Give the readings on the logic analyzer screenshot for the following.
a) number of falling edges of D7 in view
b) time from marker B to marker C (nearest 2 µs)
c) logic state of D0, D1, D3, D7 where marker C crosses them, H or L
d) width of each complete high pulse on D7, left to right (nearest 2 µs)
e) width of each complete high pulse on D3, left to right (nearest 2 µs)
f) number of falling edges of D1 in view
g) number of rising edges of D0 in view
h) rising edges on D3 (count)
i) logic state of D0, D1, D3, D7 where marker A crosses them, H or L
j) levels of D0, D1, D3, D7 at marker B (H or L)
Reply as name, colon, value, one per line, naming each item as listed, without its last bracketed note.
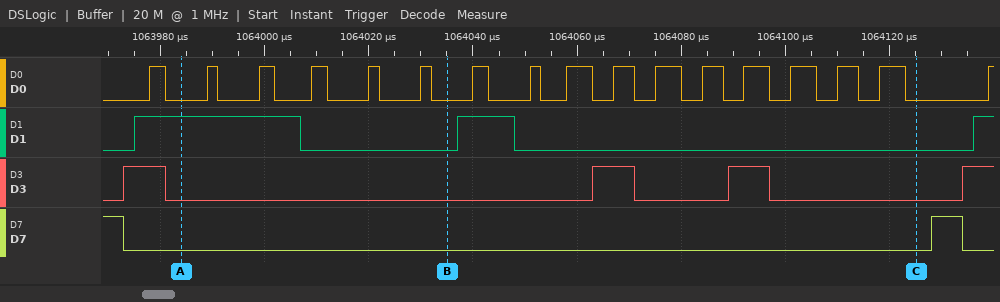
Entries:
number of falling edges of D7 in view: 2
time from marker B to marker C: 90 µs
logic state of D0, D1, D3, D7 where marker C crosses them, H or L: D0=L, D1=L, D3=L, D7=L
width of each complete high pulse on D7, left to right: 6 µs
width of each complete high pulse on D3, left to right: 8 µs, 8 µs, 8 µs
number of falling edges of D1 in view: 2
number of rising edges of D0 in view: 17
rising edges on D3: 4
logic state of D0, D1, D3, D7 where marker A crosses them, H or L: D0=L, D1=H, D3=L, D7=L
levels of D0, D1, D3, D7 at marker B: D0=L, D1=L, D3=L, D7=L
